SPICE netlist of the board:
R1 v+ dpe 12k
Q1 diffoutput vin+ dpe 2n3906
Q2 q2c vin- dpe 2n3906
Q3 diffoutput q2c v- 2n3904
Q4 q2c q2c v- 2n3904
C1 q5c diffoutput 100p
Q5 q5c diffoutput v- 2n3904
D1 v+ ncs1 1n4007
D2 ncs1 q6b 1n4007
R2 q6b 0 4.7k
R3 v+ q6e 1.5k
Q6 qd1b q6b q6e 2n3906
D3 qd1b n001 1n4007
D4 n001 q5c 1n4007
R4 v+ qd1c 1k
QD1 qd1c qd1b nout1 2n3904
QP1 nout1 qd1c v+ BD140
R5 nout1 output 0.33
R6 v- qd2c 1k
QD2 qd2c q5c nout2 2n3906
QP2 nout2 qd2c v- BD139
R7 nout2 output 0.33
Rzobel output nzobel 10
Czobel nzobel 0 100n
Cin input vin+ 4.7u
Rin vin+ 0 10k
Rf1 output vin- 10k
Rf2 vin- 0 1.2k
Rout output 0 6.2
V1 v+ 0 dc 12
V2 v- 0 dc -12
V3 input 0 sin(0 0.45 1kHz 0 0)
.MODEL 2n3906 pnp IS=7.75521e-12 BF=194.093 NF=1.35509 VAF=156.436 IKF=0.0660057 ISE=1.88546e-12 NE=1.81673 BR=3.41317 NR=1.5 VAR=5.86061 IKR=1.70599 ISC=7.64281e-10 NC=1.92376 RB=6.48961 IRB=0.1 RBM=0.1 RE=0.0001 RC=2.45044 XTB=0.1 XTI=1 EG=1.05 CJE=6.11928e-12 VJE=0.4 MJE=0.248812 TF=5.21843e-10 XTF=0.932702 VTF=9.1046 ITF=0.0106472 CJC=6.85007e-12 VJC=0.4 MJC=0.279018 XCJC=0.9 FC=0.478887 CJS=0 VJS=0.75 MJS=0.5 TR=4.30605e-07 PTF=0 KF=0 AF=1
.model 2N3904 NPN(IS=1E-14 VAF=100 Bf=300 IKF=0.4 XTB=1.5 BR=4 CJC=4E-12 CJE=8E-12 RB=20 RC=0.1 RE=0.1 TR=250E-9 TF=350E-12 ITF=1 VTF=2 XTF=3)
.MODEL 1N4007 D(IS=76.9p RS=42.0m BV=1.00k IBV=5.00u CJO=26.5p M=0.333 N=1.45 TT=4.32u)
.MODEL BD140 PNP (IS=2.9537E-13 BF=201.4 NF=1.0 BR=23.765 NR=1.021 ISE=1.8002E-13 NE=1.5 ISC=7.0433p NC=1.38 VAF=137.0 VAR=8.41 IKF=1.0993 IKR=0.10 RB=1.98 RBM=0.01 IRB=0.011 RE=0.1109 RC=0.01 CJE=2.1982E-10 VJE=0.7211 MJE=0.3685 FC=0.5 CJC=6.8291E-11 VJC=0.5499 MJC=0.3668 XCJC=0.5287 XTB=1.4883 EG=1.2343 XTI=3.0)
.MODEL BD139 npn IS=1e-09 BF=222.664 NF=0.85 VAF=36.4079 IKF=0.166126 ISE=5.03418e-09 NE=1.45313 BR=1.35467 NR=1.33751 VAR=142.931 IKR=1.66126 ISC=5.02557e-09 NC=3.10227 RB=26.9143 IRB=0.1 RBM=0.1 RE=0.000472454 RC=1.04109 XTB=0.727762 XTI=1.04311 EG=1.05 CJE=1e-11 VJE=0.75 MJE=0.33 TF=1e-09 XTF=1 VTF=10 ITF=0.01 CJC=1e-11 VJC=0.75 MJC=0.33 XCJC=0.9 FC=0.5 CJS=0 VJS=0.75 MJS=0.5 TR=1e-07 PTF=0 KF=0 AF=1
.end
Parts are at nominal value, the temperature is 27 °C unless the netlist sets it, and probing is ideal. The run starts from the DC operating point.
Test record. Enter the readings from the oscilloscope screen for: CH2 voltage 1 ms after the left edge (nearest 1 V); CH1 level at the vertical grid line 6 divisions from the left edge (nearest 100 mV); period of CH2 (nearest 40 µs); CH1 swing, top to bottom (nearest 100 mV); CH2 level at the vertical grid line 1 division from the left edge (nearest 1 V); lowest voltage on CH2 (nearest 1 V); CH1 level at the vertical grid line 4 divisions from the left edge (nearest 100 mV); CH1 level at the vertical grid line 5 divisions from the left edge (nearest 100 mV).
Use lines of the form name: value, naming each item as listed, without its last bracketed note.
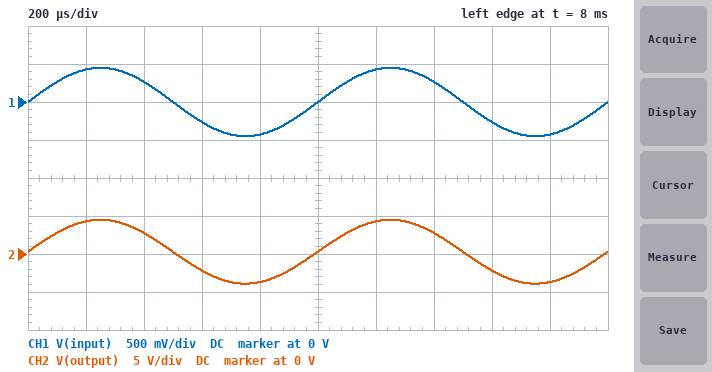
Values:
CH2 voltage 1 ms after the left edge: 0 V
CH1 level at the vertical grid line 6 divisions from the left edge: 400 mV
period of CH2: 1.00 ms
CH1 swing, top to bottom: 900 mV
CH2 level at the vertical grid line 1 division from the left edge: 4 V
lowest voltage on CH2: -4 V
CH1 level at the vertical grid line 4 divisions from the left edge: -400 mV
CH1 level at the vertical grid line 5 divisions from the left edge: 0 V
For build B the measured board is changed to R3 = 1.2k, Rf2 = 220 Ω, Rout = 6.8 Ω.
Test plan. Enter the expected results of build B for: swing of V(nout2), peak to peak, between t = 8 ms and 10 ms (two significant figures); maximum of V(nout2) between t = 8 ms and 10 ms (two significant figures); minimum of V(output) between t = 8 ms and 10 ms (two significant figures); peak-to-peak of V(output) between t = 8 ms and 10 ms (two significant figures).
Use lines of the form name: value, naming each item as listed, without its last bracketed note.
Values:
swing of V(nout2), peak to peak, between t = 8 ms and 10 ms: 21 V
maximum of V(nout2) between t = 8 ms and 10 ms: 10 V
minimum of V(output) between t = 8 ms and 10 ms: -10 V
peak-to-peak of V(output) between t = 8 ms and 10 ms: 20 V
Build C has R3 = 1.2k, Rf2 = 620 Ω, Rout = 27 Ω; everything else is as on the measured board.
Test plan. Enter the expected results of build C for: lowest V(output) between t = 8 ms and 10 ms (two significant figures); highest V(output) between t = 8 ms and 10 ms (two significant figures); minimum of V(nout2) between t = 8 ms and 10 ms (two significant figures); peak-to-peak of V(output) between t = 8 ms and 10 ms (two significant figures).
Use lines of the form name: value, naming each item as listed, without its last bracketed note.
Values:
lowest V(output) between t = 8 ms and 10 ms: -7.1 V
highest V(output) between t = 8 ms and 10 ms: 8.3 V
minimum of V(nout2) between t = 8 ms and 10 ms: -7.2 V
peak-to-peak of V(output) between t = 8 ms and 10 ms: 15 V
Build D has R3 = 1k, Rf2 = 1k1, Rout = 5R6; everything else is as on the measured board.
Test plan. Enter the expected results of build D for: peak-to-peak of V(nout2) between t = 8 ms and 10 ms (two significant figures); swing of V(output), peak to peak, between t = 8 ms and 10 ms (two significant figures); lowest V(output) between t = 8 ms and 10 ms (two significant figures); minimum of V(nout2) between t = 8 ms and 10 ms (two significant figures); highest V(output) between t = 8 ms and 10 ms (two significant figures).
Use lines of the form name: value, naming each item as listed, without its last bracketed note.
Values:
peak-to-peak of V(nout2) between t = 8 ms and 10 ms: 9.3 V
swing of V(output), peak to peak, between t = 8 ms and 10 ms: 9.1 V
lowest V(output) between t = 8 ms and 10 ms: -4.2 V
minimum of V(nout2) between t = 8 ms and 10 ms: -4.5 V
highest V(output) between t = 8 ms and 10 ms: 4.9 V
